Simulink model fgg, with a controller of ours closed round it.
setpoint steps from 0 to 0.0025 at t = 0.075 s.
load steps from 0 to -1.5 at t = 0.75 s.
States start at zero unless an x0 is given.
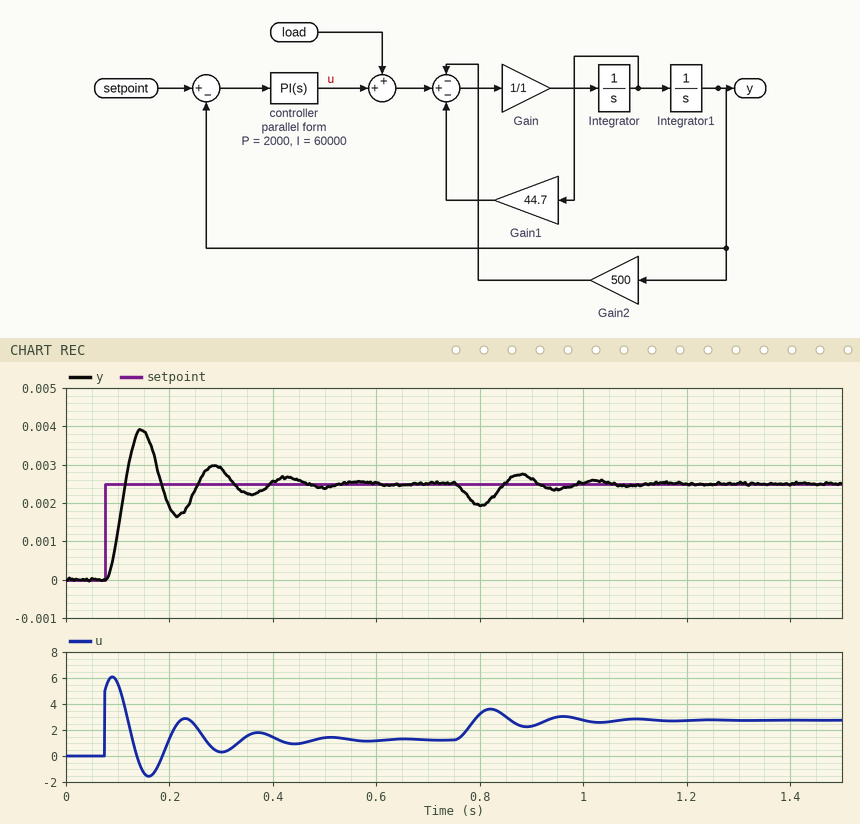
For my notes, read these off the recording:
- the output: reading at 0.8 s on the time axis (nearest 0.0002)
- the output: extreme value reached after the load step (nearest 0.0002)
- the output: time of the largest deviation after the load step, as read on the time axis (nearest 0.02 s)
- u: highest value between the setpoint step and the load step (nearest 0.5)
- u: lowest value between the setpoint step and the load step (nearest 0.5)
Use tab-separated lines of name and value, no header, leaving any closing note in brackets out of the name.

the output: reading at 0.8 s on the time axis	0.0020
the output: extreme value reached after the load step	0.0020
the output: time of the largest deviation after the load step, as read on the time axis	0.80 s
u: highest value between the setpoint step and the load step	6.0
u: lowest value between the setpoint step and the load step	-1.5
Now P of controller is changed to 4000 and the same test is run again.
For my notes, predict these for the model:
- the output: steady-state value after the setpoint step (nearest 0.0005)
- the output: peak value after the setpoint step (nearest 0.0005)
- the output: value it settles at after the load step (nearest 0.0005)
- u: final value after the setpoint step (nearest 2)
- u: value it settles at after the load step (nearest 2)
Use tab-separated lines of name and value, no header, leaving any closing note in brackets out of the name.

the output: steady-state value after the setpoint step	0.0025
the output: peak value after the setpoint step	0.0035
the output: value it settles at after the load step	0.0025
u: final value after the setpoint step	2
u: value it settles at after the load step	2
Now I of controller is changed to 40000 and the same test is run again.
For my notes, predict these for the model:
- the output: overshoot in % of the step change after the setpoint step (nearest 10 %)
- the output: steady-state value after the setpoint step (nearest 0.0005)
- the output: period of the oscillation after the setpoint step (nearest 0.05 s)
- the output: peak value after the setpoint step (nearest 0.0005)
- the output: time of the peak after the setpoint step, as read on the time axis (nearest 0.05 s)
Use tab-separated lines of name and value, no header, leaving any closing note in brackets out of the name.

the output: overshoot in % of the step change after the setpoint step	40 %
the output: steady-state value after the setpoint step	0.0025
the output: period of the oscillation after the setpoint step	0.15 s
the output: peak value after the setpoint step	0.0035
the output: time of the peak after the setpoint step, as read on the time axis	0.15 s
